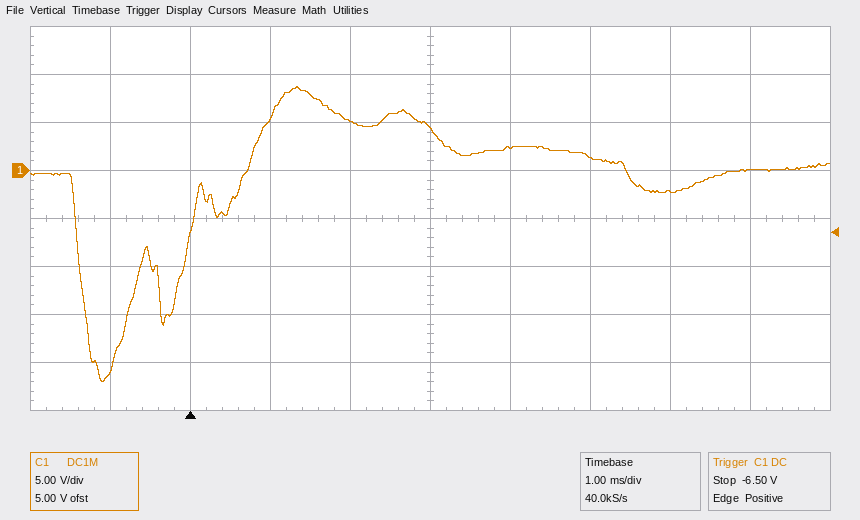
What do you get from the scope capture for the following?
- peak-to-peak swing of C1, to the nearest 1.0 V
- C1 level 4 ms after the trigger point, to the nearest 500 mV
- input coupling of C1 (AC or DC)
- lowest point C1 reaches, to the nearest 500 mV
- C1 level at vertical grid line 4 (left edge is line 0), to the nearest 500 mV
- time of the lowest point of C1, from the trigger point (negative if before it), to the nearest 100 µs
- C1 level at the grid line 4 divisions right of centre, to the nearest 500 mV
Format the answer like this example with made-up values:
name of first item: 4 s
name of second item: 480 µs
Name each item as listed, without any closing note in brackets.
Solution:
peak-to-peak swing of C1, to the nearest 1.0 V: 31.0 V
C1 level 4 ms after the trigger point, to the nearest 500 mV: 2.5 V
input coupling of C1: DC
lowest point C1 reaches, to the nearest 500 mV: -22.0 V
C1 level at vertical grid line 4 (left edge is line 0), to the nearest 500 mV: 5.0 V
time of the lowest point of C1, from the trigger point (negative if before it), to the nearest 100 µs: -1.1 ms
C1 level at the grid line 4 divisions right of centre, to the nearest 500 mV: 0.0 V
